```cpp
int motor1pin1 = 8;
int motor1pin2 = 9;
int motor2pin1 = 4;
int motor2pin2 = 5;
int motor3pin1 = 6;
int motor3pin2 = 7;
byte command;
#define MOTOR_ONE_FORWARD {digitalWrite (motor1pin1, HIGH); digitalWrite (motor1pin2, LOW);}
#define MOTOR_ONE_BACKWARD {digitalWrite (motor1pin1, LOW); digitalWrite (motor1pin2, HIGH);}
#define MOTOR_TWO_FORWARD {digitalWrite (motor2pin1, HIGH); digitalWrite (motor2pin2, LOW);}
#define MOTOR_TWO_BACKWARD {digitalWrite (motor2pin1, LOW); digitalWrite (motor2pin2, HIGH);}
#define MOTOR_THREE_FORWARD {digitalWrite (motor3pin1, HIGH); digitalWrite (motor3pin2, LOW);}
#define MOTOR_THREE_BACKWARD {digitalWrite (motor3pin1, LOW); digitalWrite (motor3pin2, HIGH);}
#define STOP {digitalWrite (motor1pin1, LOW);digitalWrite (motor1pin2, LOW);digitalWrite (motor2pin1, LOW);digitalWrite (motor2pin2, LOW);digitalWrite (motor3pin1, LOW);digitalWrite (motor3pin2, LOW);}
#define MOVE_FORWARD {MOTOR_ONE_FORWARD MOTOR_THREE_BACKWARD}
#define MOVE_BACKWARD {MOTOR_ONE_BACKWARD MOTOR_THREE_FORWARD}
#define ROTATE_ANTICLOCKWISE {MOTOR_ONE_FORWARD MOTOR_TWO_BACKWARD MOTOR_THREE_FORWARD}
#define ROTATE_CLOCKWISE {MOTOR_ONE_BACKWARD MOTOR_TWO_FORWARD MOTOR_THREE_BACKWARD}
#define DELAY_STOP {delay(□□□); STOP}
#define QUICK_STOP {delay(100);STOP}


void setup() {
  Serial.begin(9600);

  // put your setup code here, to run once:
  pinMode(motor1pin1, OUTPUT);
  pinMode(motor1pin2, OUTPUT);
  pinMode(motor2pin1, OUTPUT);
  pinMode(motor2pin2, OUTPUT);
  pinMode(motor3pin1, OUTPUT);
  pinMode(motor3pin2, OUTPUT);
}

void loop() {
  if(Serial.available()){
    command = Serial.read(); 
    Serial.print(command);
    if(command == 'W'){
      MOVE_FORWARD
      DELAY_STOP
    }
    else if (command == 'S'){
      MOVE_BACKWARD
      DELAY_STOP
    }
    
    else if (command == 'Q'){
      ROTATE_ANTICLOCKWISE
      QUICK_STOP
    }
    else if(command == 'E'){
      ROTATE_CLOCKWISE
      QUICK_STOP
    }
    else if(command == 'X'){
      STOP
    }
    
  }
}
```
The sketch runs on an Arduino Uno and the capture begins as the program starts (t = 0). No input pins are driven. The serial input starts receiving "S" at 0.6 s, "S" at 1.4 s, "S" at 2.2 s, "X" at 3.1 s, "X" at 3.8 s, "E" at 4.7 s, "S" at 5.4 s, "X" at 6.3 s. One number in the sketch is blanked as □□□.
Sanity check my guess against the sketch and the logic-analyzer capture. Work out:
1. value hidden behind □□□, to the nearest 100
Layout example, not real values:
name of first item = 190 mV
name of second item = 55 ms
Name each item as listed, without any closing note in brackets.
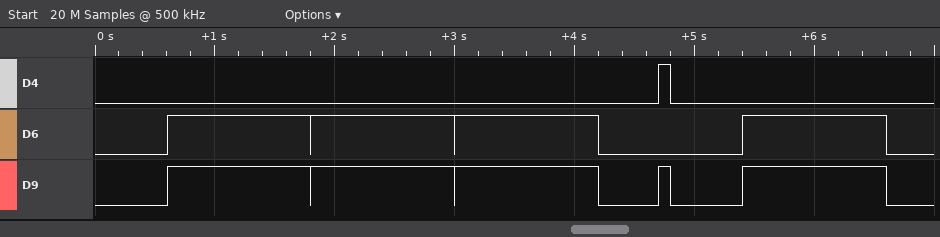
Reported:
value hidden behind □□□, to the nearest 100 = 1200
